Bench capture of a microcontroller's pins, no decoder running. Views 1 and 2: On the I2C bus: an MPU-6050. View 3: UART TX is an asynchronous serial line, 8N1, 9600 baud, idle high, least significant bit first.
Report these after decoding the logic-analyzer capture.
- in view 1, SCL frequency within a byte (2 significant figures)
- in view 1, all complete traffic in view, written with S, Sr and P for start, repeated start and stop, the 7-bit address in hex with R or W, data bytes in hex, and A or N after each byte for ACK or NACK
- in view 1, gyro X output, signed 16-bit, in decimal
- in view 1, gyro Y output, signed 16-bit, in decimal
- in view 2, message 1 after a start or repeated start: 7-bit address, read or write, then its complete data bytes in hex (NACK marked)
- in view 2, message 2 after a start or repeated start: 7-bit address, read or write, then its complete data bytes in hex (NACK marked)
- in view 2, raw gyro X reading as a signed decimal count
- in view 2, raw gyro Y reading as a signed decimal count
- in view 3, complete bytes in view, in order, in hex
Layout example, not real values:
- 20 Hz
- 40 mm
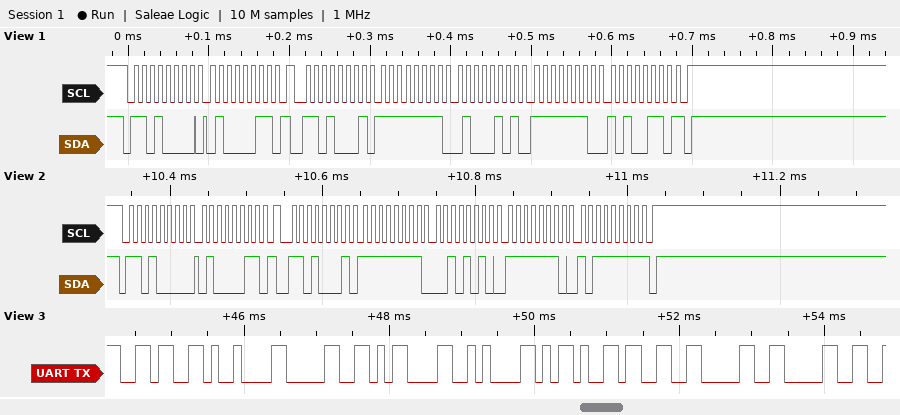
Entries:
- 100 kHz
- S 68W A 43 A Sr 68R A FF A 45 A FE A A6 N P
- -187
- -346
- 0x68 write: 43
- 0x68 read: FF 2A FE BF NACK
- -214
- -321
- 36 09 30 0D 0A 2D 33 30 30
